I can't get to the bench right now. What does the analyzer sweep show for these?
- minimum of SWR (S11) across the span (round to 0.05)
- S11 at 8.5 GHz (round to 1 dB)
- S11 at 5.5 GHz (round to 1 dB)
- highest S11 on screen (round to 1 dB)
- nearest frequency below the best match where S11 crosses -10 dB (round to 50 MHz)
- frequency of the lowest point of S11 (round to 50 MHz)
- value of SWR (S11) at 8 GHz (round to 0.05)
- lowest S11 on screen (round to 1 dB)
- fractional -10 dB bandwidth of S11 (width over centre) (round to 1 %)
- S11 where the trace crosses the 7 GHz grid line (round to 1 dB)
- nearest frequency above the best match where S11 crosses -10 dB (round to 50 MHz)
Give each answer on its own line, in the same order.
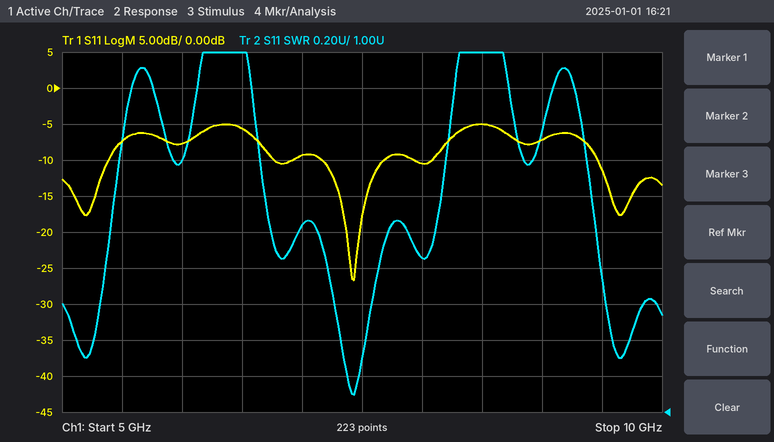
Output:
1.10
-5 dB
-7 dB
-5 dB
7.15 GHz
7.45 GHz
1.85
-27 dB
7 %
-9 dB
7.70 GHz
